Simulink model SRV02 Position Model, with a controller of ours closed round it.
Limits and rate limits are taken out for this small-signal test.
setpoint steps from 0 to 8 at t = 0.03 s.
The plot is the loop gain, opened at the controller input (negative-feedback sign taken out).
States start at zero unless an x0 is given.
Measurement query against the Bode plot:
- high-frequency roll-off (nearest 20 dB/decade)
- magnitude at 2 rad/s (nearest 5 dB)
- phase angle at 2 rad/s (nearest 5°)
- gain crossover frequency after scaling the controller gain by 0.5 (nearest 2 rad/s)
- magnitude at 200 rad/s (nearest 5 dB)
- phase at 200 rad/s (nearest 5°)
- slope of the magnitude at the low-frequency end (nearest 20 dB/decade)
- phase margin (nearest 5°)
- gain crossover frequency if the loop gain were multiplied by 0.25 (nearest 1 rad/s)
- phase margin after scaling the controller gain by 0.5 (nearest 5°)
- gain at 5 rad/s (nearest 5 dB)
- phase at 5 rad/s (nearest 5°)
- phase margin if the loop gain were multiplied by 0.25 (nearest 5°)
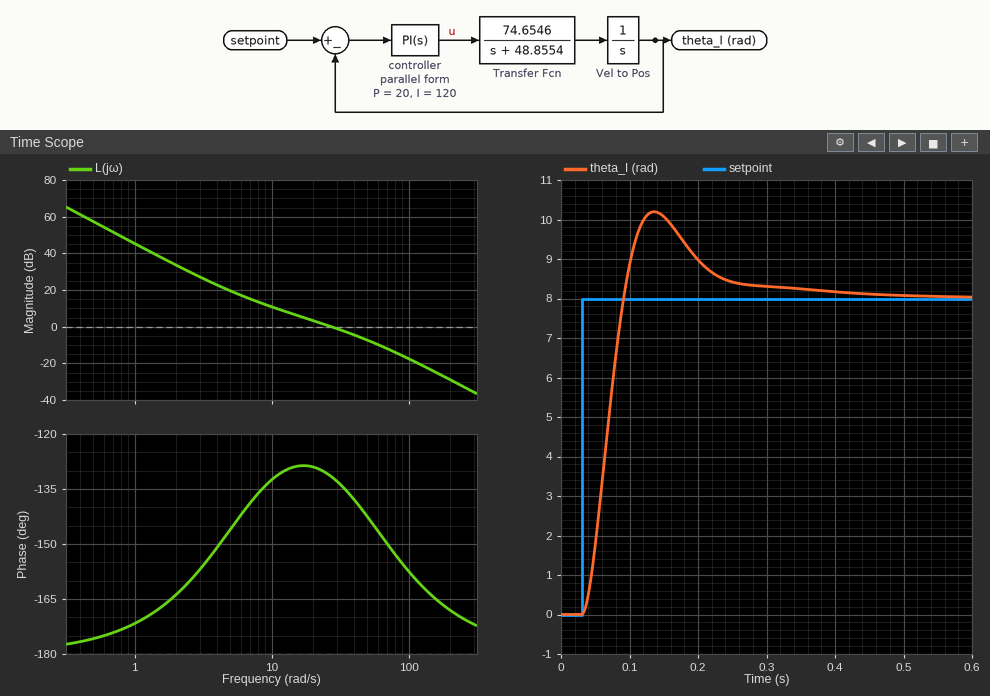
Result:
-40 dB/decade
35 dB
-165°
16 rad/s
-30 dB
-170°
-40 dB/decade
50°
9 rad/s
50°
20 dB
-145°
45°
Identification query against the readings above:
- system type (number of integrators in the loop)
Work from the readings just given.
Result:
2
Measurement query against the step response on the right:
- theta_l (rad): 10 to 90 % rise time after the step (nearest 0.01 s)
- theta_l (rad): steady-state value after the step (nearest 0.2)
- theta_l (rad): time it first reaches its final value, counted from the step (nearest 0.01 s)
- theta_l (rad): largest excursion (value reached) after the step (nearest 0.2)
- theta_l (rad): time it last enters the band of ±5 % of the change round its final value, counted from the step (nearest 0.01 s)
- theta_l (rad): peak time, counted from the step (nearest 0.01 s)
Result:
0.04 s
8.0
0.06 s
10.2
0.22 s
0.11 s
